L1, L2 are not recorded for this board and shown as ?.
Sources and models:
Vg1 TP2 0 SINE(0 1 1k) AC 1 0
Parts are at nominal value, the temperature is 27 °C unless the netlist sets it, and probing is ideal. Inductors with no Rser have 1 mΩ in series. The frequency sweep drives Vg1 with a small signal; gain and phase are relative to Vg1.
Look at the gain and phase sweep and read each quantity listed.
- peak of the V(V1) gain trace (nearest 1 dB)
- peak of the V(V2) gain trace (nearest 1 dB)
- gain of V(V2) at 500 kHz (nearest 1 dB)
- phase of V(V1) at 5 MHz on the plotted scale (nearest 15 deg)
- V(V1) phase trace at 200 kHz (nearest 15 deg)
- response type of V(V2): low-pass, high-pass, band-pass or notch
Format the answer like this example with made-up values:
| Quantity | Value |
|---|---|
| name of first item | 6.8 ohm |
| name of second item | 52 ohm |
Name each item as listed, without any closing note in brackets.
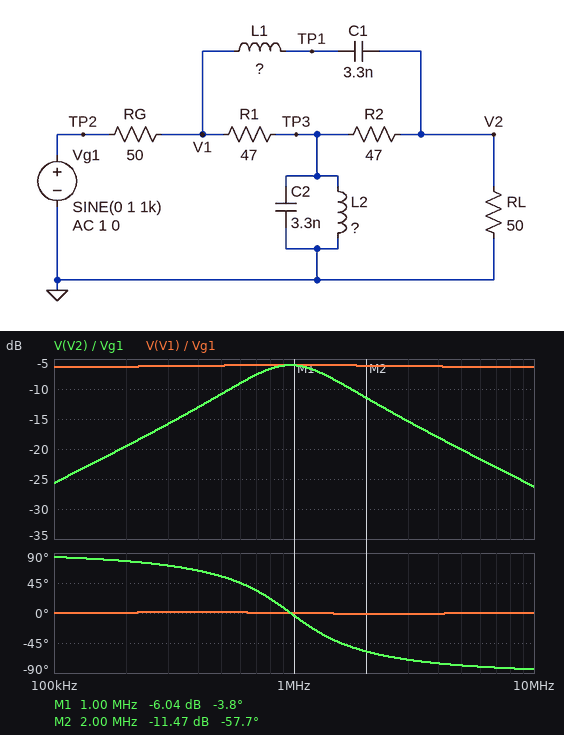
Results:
| Quantity | Value |
|---|---|
| peak of the V(V1) gain trace | -6 dB |
| peak of the V(V2) gain trace | -6 dB |
| gain of V(V2) at 500 kHz | -11 dB |
| phase of V(V1) at 5 MHz on the plotted scale | 0 deg |
| V(V1) phase trace at 200 kHz | 0 deg |
| response type of V(V2): low-pass, high-pass, band-pass or notch | band-pass |
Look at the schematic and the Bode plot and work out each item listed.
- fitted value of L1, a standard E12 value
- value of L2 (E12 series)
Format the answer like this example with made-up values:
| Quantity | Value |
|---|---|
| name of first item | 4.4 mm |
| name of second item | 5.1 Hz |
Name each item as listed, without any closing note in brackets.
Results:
| Quantity | Value |
|---|---|
| fitted value of L1, a standard E12 value | 8.2 µH |
| value of L2 | 8.2 µH |
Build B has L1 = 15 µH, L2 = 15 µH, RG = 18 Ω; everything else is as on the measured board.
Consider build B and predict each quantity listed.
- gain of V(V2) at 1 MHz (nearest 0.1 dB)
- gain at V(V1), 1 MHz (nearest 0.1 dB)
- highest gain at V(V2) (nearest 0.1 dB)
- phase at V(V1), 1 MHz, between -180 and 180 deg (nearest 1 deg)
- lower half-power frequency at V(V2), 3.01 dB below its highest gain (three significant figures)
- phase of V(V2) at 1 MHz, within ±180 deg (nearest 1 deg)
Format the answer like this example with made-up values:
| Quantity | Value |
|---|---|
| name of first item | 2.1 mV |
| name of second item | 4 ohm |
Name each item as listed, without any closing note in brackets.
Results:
| Quantity | Value |
|---|---|
| gain of V(V2) at 1 MHz | -5.1 dB |
| gain at V(V1), 1 MHz | -2.1 dB |
| highest gain at V(V2) | -2.7 dB |
| phase at V(V1), 1 MHz, between -180 and 180 deg | 1 deg |
| lower half-power frequency at V(V2), 3.01 dB below its highest gain | 480 kHz |
| phase of V(V2) at 1 MHz, within ±180 deg | -35 deg |
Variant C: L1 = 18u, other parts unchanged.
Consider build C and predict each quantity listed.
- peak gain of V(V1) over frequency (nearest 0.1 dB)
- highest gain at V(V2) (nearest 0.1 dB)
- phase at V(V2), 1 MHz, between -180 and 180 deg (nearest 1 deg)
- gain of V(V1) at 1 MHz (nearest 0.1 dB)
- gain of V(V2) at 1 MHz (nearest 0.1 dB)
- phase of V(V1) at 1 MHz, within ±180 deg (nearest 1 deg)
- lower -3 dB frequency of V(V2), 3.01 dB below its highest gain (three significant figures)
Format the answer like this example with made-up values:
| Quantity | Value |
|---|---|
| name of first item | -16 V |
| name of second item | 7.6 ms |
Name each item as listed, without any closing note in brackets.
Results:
| Quantity | Value |
|---|---|
| peak gain of V(V1) over frequency | -3.5 dB |
| highest gain at V(V2) | -7.5 dB |
| phase at V(V2), 1 MHz, between -180 and 180 deg | -21 deg |
| gain of V(V1) at 1 MHz | -3.6 dB |
| gain of V(V2) at 1 MHz | -8.7 dB |
| phase of V(V1) at 1 MHz, within ±180 deg | 9 deg |
| lower -3 dB frequency of V(V2), 3.01 dB below its highest gain | 458 kHz |
